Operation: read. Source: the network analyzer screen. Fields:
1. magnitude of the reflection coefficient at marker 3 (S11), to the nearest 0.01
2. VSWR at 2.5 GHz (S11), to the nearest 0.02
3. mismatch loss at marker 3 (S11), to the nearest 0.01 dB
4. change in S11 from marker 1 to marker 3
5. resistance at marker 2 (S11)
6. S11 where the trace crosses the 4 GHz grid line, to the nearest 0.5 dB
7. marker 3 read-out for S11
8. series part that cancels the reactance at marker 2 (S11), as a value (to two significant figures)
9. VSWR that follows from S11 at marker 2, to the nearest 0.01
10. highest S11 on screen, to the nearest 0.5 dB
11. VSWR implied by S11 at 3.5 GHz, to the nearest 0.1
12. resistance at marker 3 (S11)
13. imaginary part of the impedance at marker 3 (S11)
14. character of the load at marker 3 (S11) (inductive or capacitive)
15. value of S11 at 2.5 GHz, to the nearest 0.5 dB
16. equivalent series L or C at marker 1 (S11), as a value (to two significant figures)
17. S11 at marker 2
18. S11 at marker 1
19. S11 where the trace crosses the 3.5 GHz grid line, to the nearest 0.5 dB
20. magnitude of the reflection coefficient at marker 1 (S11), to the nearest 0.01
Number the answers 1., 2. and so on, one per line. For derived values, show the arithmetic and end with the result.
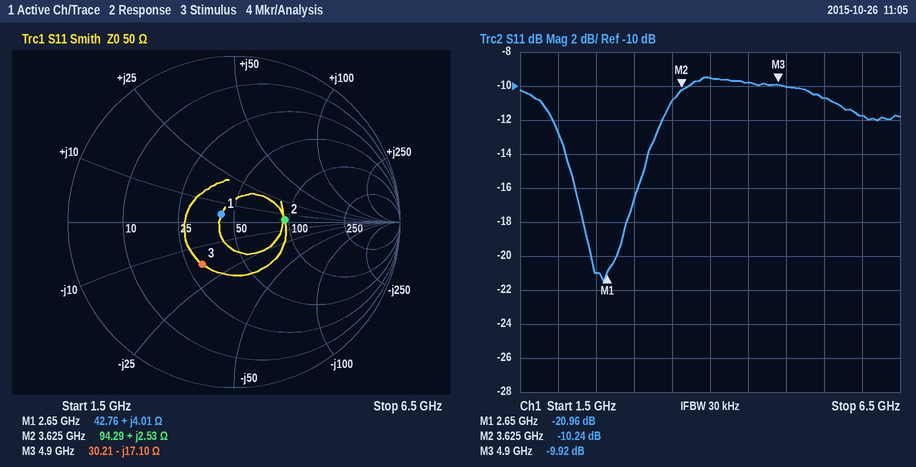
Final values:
1. 0.32
2. |Γ| = 10^(-21/20) = 0.0891; VSWR = (1 + 0.0891)/(1 − 0.0891) ≈ 1.20
3. −10 log10(1 − 10^(-9.92/10)) ≈ 0.47 dB
4. -9.92 − (-20.96) = 11.04 dB
5. 94.29 Ω
6. -9.5 dB
7. -9.92 dB
8. C = 1/(2π × 3.625 GHz × 2.53 Ω) ≈ 17 pF
9. (1 + 0.3076)/(1 − 0.3076) ≈ 1.89
10. -9.5 dB
11. |Γ| = 10^(-11/20) = 0.2818; VSWR = (1 + 0.2818)/(1 − 0.2818) ≈ 1.8
12. 30.21 Ω
13. -17.10 Ω
14. capacitive
15. -21.0 dB
16. L = 4.01 Ω/(2π × 2.65 GHz) ≈ 241 pH, so 240 pH to two significant figures
17. -10.24 dB
18. -20.96 dB
19. -11.0 dB
20. 0.09
